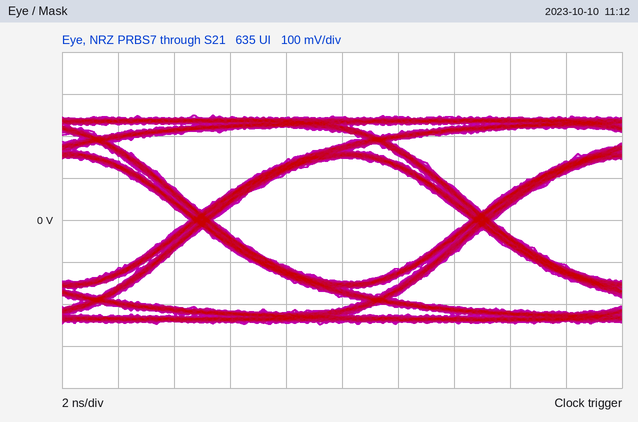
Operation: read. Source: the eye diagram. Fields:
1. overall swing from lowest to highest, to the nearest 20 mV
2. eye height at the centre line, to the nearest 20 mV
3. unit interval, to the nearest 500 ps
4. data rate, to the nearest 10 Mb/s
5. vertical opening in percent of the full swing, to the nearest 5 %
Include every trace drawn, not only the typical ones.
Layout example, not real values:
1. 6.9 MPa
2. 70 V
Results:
1. 500 mV
2. 300 mV
3. 10.0 ns
4. 100 Mb/s
5. 60 %
